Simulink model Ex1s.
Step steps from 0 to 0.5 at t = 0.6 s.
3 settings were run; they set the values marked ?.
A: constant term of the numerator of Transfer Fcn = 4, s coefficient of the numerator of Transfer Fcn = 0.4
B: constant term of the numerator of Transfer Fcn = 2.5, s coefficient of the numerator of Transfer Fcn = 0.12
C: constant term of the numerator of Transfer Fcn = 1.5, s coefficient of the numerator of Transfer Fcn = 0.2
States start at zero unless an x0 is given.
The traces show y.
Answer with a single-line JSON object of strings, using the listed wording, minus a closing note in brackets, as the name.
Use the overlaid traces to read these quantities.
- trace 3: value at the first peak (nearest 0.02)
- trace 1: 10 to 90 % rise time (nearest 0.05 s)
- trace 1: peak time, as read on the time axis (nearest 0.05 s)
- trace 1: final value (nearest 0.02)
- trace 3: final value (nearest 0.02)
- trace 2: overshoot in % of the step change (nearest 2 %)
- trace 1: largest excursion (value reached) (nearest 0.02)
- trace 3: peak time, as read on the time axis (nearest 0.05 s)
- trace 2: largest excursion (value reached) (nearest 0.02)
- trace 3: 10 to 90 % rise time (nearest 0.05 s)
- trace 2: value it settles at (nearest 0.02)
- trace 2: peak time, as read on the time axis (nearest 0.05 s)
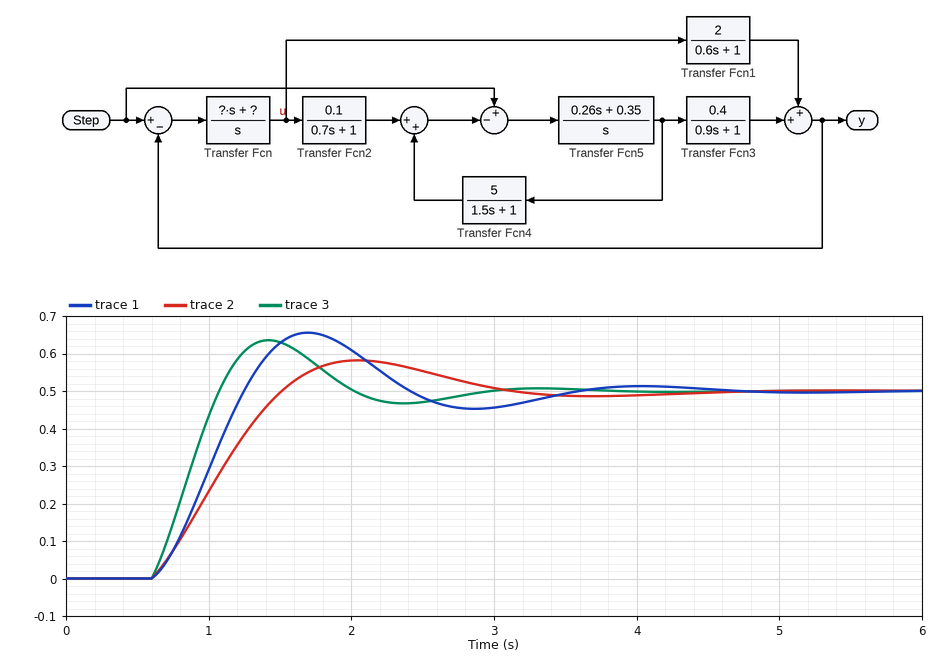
{"trace 3: value at the first peak": "0.64", "trace 1: 10 to 90 % rise time": "0.45 s", "trace 1: peak time, as read on the time axis": "1.70 s", "trace 1: final value": "0.50", "trace 3: final value": "0.50", "trace 2: overshoot in % of the step change": "16 %", "trace 1: largest excursion (value reached)": "0.66", "trace 3: peak time, as read on the time axis": "1.40 s", "trace 2: largest excursion (value reached)": "0.58", "trace 3: 10 to 90 % rise time": "0.35 s", "trace 2: value it settles at": "0.50", "trace 2: peak time, as read on the time axis": "2.05 s"}
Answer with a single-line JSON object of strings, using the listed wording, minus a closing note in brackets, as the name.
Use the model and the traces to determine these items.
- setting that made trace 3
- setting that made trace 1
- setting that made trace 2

{"setting that made trace 3": "A", "setting that made trace 1": "B", "setting that made trace 2": "C"}
